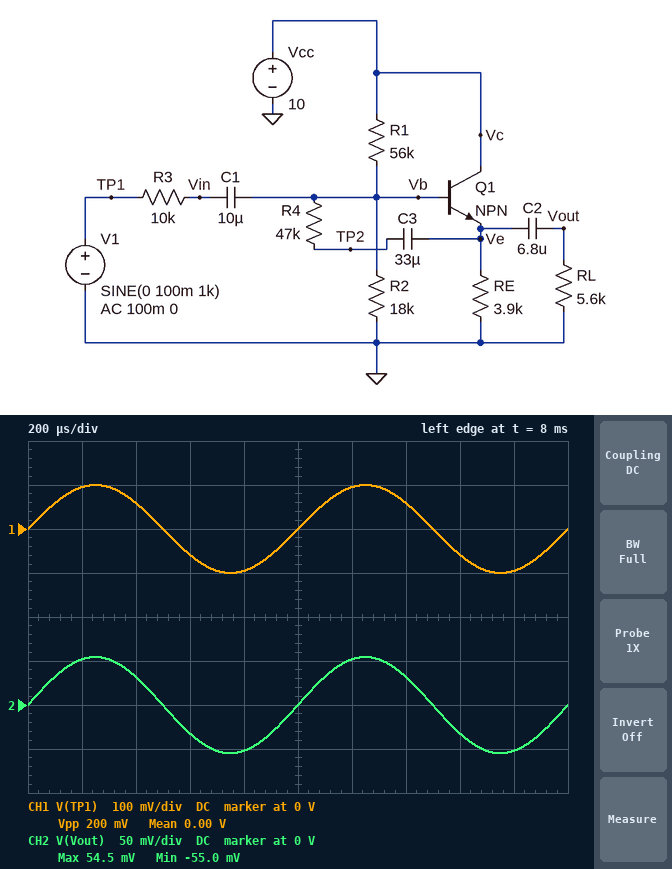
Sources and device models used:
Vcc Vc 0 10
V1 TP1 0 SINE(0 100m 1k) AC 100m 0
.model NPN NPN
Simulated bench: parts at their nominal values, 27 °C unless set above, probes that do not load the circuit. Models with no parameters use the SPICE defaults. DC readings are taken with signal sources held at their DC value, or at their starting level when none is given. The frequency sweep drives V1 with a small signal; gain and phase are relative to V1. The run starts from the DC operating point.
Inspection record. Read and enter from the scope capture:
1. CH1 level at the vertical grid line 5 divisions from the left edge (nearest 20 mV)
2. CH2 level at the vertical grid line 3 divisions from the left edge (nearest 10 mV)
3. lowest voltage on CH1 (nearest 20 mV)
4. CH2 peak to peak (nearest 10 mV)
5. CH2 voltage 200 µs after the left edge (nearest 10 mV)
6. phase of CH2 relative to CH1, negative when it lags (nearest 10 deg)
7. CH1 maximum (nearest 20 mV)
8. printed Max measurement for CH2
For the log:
0 V
-30 mV
-100 mV
110 mV
50 mV
0 deg
100 mV
54.5 mV
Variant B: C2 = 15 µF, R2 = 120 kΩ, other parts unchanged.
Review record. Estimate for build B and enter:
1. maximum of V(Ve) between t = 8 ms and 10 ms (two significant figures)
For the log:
5.6 V
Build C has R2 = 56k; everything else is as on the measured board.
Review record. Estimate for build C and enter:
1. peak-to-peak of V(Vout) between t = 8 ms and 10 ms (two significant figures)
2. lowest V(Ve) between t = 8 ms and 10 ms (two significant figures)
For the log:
140 mV
3.9 V
